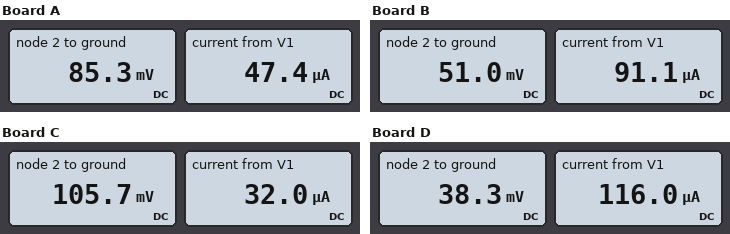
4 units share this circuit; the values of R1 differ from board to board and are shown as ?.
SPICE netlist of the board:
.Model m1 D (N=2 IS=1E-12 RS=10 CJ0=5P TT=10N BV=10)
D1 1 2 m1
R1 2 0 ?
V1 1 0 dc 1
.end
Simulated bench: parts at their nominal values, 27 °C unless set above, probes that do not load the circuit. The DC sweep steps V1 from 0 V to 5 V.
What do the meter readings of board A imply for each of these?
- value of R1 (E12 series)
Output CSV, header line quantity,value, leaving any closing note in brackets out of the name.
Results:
quantity,value
value of R1,1.8 kΩ
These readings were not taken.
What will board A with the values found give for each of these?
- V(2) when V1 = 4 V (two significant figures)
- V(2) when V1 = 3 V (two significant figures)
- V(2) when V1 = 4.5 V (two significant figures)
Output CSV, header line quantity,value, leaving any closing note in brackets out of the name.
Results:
quantity,value
V(2) when V1 = 4 V,2.9 V
V(2) when V1 = 3 V,1.9 V
V(2) when V1 = 4.5 V,3.4 V
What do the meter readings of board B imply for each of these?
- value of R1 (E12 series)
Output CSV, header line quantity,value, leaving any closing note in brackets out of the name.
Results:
quantity,value
value of R1,560 Ω
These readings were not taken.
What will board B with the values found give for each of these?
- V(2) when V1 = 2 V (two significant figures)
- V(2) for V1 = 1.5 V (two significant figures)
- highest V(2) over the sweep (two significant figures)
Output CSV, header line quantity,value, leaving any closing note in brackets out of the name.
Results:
quantity,value
V(2) when V1 = 2 V,890 mV
V(2) for V1 = 1.5 V,430 mV
highest V(2) over the sweep,3.8 V
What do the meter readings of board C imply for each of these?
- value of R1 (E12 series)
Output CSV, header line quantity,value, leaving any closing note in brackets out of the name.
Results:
quantity,value
value of R1,3.3 kΩ
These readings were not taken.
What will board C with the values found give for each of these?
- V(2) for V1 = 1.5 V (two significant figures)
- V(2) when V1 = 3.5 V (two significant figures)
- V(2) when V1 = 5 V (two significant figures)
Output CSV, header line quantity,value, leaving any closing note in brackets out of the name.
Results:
quantity,value
V(2) for V1 = 1.5 V,520 mV
V(2) when V1 = 3.5 V,2.4 V
V(2) when V1 = 5 V,3.9 V
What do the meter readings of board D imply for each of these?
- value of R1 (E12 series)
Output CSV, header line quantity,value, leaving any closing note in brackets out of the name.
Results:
quantity,value
value of R1,330 Ω
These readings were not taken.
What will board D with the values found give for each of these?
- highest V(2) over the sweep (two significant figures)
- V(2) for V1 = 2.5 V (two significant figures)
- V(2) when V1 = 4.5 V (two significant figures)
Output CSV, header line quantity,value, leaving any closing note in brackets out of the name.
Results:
quantity,value
highest V(2) over the sweep,3.7 V
V(2) for V1 = 2.5 V,1.3 V
V(2) when V1 = 4.5 V,3.2 V
